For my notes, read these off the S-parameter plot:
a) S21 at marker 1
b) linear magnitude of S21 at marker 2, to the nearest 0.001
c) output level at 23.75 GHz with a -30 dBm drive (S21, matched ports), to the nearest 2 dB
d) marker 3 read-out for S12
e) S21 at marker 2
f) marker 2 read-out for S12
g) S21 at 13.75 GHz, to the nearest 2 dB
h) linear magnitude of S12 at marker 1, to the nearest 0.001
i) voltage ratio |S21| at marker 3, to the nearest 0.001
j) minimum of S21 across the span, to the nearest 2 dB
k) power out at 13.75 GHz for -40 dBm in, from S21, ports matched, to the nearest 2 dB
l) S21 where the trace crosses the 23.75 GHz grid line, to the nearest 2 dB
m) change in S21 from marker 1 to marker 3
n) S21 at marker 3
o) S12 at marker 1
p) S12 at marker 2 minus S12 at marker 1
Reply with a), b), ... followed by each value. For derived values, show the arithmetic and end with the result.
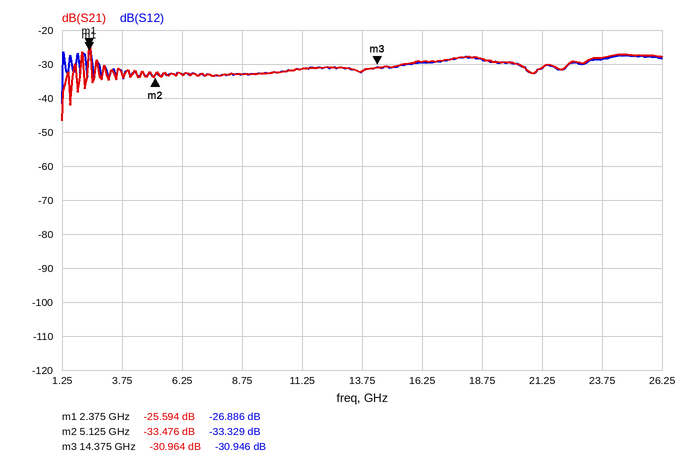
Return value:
a) -25.594 dB
b) 10^(-33.476/20) ≈ 0.021
c) -30 dBm + (-28 dB) = -58 dBm
d) -30.946 dB
e) -33.476 dB
f) -33.329 dB
g) -32 dB
h) 10^(-26.886/20) ≈ 0.045
i) 10^(-30.964/20) ≈ 0.028
j) -46 dB
k) -40 dBm + (-32 dB) = -72 dBm
l) -28 dB
m) -30.964 − (-25.594) = -5.370 dB
n) -30.964 dB
o) -26.886 dB
p) -33.329 − (-26.886) = -6.443 dB
